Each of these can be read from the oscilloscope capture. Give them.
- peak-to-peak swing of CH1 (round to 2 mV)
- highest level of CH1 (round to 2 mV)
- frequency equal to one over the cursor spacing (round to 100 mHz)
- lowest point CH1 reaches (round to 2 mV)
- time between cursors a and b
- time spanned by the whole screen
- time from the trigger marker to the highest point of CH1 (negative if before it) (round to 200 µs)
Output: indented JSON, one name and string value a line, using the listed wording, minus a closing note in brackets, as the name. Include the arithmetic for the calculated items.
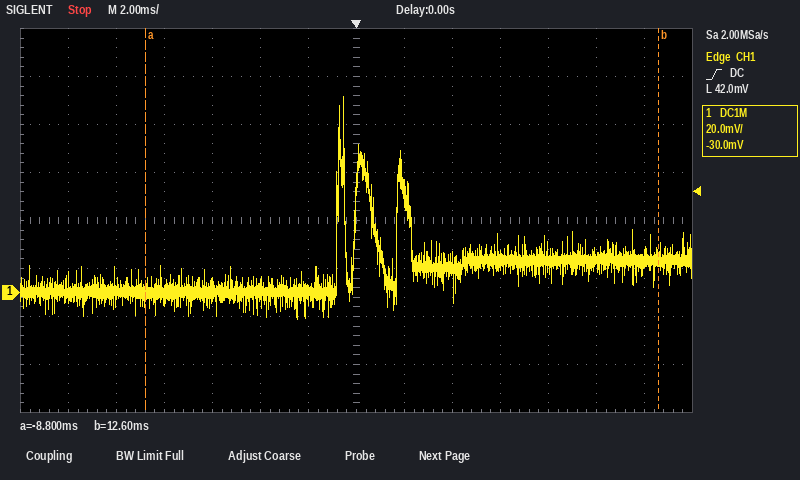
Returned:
{
  "peak-to-peak swing of CH1": "82 mV − (-10 mV) = 92 mV",
  "highest level of CH1": "82 mV",
  "frequency equal to one over the cursor spacing": "1 / 21.4 ms ≈ 46.7 Hz",
  "lowest point CH1 reaches": "-10 mV",
  "time between cursors a and b": "12.6 ms − (-8.8 ms) = 21.4 ms",
  "time spanned by the whole screen": "28 ms",
  "time from the trigger marker to the highest point of CH1 (negative if before it)": "-600 µs"
}
